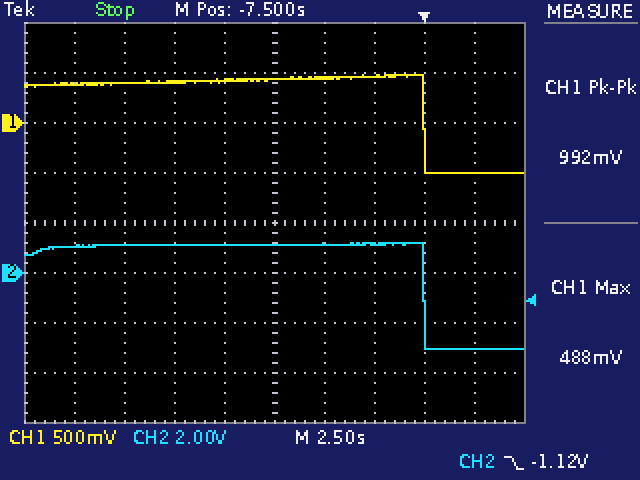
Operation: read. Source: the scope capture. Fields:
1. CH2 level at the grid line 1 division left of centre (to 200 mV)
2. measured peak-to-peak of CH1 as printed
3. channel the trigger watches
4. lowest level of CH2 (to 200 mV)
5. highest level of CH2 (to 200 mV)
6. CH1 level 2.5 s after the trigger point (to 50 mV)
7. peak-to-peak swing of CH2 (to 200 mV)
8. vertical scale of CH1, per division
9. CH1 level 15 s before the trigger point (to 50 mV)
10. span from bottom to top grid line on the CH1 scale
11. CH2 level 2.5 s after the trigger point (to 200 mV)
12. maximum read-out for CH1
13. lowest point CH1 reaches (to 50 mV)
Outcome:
1.2 V
992 mV
CH2
-3.0 V
1.2 V
-500 mV
4.2 V
500 mV
400 mV
4 V
-3.0 V
488 mV
-500 mV
